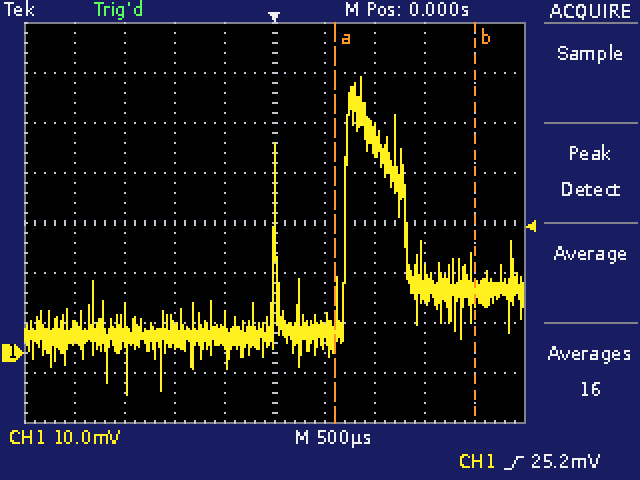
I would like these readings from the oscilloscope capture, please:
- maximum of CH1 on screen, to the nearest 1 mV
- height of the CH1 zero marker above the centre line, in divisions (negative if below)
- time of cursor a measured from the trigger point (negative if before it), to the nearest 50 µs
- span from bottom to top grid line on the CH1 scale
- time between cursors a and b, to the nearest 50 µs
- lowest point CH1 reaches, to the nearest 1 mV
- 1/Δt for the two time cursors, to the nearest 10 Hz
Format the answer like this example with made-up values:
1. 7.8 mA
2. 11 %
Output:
1. 55 mV
2. -2.6 div
3. +600 µs
4. 80 mV
5. 1.40 ms
6. -8 mV
7. 710 Hz
